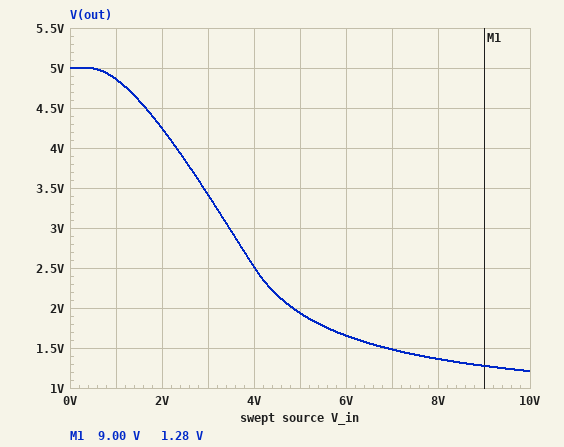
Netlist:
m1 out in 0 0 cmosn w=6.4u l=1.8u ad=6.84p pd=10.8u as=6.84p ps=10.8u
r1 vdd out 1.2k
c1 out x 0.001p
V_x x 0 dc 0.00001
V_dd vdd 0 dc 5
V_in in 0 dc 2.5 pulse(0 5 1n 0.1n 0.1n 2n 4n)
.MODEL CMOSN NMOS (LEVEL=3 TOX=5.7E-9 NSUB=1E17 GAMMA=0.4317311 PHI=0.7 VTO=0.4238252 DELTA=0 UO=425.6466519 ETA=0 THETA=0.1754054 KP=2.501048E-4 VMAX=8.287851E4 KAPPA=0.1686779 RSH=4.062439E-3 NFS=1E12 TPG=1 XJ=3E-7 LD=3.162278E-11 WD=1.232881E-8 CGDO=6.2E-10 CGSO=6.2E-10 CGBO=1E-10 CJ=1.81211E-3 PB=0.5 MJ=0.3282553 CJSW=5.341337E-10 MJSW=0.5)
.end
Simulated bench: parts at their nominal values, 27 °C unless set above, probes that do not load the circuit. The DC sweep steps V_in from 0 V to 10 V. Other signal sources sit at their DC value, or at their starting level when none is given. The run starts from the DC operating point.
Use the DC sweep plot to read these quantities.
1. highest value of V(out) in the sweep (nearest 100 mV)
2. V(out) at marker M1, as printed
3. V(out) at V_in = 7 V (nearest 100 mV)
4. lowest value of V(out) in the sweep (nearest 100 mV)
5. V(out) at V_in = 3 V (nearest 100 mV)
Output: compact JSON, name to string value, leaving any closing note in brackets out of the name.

{"highest value of V(out) in the sweep": "5.0 V", "V(out) at marker M1, as printed": "1.28 V", "V(out) at V_in = 7 V": "1.5 V", "lowest value of V(out) in the sweep": "1.2 V", "V(out) at V_in = 3 V": "3.4 V"}
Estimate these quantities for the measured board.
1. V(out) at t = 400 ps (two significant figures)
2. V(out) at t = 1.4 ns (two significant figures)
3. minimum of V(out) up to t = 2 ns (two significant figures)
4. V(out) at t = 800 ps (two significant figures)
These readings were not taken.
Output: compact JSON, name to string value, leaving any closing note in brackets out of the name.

{"V(out) at t = 400 ps": "5.0 V", "V(out) at t = 1.4 ns": "1.9 V", "minimum of V(out) up to t = 2 ns": "1.9 V", "V(out) at t = 800 ps": "5.0 V"}
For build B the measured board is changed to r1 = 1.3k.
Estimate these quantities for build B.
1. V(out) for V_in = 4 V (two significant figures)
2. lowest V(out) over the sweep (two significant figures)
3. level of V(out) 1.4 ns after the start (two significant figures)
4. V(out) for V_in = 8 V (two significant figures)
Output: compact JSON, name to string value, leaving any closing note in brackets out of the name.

{"V(out) for V_in = 4 V": "2.3 V", "lowest V(out) over the sweep": "1.1 V", "level of V(out) 1.4 ns after the start": "1.8 V", "V(out) for V_in = 8 V": "1.3 V"}
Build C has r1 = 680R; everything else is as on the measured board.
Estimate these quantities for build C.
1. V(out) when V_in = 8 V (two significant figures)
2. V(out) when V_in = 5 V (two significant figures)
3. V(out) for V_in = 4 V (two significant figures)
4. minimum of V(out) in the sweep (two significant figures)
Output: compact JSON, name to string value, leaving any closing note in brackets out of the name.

{"V(out) when V_in = 8 V": "2.2 V", "V(out) when V_in = 5 V": "3.0 V", "V(out) for V_in = 4 V": "3.6 V", "minimum of V(out) in the sweep": "1.9 V"}
